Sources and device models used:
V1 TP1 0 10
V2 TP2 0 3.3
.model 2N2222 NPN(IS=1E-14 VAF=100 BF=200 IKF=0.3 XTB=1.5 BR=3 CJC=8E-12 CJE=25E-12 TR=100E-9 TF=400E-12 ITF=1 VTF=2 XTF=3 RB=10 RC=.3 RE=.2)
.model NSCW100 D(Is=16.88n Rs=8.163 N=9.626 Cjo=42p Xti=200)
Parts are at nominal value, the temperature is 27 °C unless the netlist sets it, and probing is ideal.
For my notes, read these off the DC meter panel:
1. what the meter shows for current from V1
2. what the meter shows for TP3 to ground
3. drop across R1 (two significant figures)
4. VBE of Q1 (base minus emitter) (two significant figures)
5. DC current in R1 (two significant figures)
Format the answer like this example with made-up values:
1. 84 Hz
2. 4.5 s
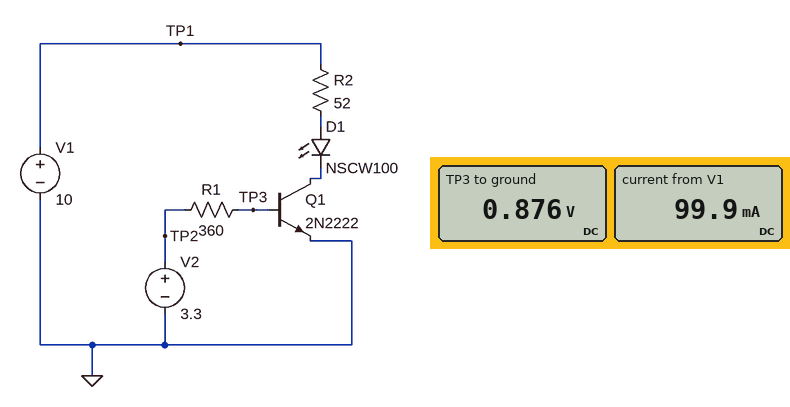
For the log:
1. 99.9 mA
2. 0.876 V
3. 2.4 V
4. 880 mV
5. 6.7 mA
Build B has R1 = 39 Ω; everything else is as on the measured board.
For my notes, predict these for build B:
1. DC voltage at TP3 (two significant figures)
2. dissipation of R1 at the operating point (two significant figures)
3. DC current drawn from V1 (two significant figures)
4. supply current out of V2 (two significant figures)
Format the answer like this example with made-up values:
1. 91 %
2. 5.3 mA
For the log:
1. 1.3 V
2. 98 mW
3. 100 mA
4. 50 mA
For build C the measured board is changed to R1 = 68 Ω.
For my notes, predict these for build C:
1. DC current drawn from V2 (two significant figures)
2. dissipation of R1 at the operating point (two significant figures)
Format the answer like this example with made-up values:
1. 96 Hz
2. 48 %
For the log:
1. 32 mA
2. 68 mW
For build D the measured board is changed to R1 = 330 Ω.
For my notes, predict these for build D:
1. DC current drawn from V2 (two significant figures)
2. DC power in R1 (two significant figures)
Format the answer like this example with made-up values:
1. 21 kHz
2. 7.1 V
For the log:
1. 7.3 mA
2. 18 mW
